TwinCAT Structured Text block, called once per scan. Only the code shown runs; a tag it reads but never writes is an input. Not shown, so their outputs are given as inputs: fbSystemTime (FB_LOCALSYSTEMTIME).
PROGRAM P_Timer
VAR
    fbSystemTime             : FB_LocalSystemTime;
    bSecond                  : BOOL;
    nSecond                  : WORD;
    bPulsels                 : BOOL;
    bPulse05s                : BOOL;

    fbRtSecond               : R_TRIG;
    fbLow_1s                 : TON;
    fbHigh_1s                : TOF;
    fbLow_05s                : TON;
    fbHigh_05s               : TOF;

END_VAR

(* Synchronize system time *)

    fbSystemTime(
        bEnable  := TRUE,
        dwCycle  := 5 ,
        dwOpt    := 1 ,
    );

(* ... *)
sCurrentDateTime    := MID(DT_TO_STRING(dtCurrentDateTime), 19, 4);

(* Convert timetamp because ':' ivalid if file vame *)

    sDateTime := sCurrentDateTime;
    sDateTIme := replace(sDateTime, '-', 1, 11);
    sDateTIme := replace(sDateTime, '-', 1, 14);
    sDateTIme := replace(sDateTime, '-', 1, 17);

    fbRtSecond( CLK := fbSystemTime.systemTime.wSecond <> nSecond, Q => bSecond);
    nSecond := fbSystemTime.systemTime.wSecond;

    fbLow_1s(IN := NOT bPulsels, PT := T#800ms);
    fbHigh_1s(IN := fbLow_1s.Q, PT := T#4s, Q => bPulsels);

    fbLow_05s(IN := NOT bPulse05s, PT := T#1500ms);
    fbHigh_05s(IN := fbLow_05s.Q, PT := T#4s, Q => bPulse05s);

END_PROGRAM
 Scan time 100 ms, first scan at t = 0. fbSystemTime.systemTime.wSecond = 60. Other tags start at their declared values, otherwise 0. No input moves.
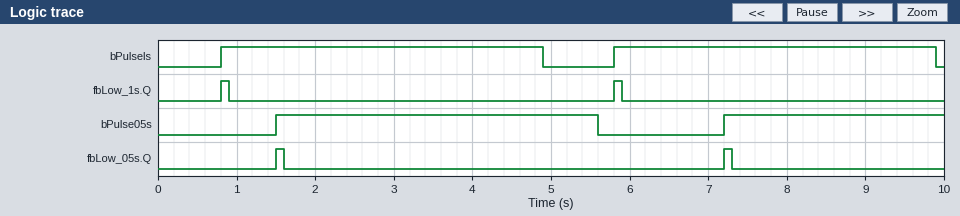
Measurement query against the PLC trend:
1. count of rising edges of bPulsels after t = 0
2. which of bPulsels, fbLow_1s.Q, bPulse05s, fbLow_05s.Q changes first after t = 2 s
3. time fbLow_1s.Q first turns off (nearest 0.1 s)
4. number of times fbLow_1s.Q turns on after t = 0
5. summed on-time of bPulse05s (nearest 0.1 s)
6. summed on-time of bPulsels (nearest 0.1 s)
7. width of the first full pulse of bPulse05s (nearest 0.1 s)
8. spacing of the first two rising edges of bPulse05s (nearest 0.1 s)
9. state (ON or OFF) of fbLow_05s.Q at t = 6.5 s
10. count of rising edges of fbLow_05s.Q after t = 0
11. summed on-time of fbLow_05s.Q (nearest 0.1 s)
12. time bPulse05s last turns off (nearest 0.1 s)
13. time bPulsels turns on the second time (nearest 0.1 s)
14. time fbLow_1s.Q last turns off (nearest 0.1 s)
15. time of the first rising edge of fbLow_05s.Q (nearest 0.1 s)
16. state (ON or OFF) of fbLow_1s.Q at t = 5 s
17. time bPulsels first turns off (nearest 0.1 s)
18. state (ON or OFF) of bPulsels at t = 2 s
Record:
2
bPulsels
0.9 s
2
6.9 s
8.2 s
4.1 s
5.7 s
OFF
2
0.2 s
5.6 s
5.8 s
5.9 s
1.5 s
OFF
4.9 s
ON
